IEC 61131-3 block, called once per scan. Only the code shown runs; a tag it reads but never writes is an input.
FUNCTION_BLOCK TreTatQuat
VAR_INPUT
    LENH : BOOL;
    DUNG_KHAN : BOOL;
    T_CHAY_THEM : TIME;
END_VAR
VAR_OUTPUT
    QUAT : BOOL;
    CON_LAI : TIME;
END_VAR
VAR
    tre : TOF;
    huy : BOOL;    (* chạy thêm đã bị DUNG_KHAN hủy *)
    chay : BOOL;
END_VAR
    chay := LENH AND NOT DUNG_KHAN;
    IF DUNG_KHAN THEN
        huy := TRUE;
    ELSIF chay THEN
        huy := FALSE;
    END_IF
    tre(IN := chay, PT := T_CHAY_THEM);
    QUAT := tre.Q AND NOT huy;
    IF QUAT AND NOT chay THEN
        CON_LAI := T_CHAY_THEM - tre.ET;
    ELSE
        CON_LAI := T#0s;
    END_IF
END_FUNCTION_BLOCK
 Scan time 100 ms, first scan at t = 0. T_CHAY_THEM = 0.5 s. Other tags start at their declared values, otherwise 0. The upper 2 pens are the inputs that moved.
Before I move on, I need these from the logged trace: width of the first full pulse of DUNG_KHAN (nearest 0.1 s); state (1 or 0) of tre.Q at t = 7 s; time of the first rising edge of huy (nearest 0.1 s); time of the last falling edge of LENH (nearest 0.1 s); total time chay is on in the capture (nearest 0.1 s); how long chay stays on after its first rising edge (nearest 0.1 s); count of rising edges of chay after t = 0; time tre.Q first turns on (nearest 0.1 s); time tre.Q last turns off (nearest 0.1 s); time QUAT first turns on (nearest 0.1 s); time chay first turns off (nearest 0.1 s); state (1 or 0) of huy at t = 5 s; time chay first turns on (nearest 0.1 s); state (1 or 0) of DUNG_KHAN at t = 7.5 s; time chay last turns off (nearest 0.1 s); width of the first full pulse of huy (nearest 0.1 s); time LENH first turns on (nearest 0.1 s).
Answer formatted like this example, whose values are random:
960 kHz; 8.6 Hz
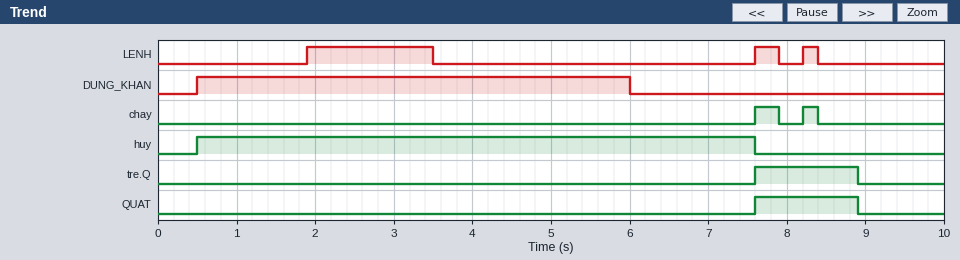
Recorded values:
5.5 s; 0; 0.5 s; 8.4 s; 0.5 s; 0.3 s; 2; 7.6 s; 8.9 s; 7.6 s; 7.9 s; 1; 7.6 s; 0; 8.4 s; 7.1 s; 1.9 s
